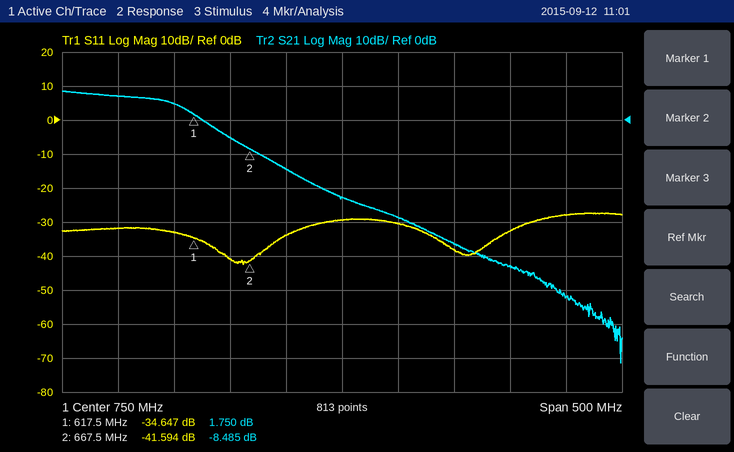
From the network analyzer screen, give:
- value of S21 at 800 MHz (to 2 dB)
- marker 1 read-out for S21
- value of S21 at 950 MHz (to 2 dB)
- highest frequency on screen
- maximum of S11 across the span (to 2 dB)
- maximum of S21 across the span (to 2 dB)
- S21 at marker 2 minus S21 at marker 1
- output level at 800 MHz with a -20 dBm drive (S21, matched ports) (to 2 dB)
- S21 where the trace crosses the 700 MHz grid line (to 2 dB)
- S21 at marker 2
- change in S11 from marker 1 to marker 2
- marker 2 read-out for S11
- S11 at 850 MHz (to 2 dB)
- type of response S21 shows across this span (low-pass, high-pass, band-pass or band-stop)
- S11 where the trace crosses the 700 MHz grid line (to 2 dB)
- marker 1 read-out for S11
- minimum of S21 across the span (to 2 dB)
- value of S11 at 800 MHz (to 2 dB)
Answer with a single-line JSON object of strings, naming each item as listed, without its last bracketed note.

{"value of S21 at 800 MHz": "-28 dB", "marker 1 read-out for S21": "1.750 dB", "value of S21 at 950 MHz": "-52 dB", "highest frequency on screen": "1 GHz", "maximum of S11 across the span": "-28 dB", "maximum of S21 across the span": "8 dB", "S21 at marker 2 minus S21 at marker 1": "-10.235 dB", "output level at 800 MHz with a -20 dBm drive (S21, matched ports)": "-48 dBm", "S21 where the trace crosses the 700 MHz grid line": "-14 dB", "S21 at marker 2": "-8.485 dB", "change in S11 from marker 1 to marker 2": "-6.947 dB", "marker 2 read-out for S11": "-41.594 dB", "S11 at 850 MHz": "-38 dB", "type of response S21 shows across this span": "low-pass", "S11 where the trace crosses the 700 MHz grid line": "-34 dB", "marker 1 read-out for S11": "-34.647 dB", "minimum of S21 across the span": "-72 dB", "value of S11 at 800 MHz": "-30 dB"}
